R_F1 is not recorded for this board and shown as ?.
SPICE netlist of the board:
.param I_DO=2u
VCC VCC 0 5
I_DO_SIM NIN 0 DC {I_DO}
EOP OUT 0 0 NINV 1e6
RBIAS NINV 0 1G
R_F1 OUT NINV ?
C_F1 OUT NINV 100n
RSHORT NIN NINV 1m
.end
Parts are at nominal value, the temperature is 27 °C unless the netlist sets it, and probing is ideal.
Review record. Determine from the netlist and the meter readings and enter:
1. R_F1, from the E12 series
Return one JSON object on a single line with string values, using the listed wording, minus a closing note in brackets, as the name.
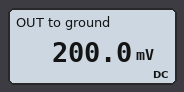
{"R_F1, from the E12 series": "100 kΩ"}
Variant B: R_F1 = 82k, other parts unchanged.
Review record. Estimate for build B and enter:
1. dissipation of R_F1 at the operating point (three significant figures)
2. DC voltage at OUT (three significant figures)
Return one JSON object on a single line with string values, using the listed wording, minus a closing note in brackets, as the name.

{"dissipation of R_F1 at the operating point": "328 nW", "DC voltage at OUT": "164 mV"}
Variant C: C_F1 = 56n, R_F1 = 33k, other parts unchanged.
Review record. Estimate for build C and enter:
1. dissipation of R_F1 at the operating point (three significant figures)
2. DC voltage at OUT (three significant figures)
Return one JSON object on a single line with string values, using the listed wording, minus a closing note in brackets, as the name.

{"dissipation of R_F1 at the operating point": "132 nW", "DC voltage at OUT": "66.0 mV"}
